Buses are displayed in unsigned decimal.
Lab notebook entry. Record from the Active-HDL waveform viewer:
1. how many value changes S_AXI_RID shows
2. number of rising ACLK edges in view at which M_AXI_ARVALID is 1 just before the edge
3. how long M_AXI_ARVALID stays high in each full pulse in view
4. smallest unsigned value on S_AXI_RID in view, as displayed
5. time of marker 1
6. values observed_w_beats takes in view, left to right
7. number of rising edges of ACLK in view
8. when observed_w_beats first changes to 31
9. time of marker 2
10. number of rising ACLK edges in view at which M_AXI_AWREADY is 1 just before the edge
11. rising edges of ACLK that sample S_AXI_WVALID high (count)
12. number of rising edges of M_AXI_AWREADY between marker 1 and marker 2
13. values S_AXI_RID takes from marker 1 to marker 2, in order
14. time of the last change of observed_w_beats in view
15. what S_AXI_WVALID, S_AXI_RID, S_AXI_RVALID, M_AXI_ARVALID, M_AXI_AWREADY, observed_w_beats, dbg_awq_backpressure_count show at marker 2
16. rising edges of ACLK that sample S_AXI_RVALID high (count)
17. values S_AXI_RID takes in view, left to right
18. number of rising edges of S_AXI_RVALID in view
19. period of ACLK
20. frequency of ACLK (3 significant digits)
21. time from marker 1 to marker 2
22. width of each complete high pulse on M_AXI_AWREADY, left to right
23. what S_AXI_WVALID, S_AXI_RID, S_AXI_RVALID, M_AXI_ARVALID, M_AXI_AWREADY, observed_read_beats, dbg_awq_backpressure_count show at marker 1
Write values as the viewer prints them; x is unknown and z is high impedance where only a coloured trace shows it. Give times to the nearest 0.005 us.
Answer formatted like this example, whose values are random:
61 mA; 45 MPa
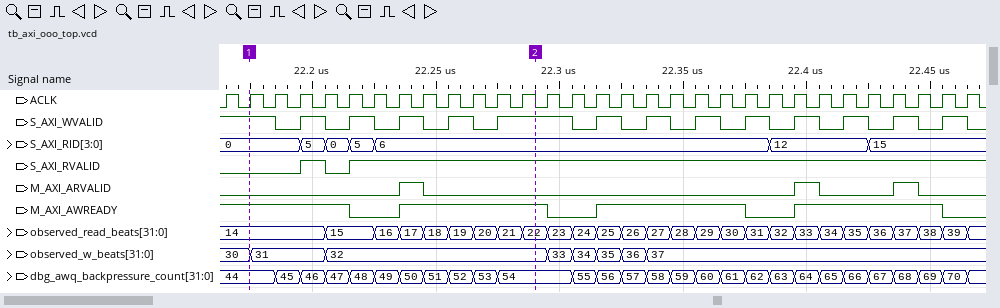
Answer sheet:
6; 3; 0.01 us, 0.01 us, 0.01 us; 0; 22.175 us; 30, 31, 32, 33, 34, 35, 36, 37; 31; 22.175 us; 22.29 us; 24; 18; 1; 0, 5, 0, 5, 6; 22.335 us; S_AXI_WVALID=1, S_AXI_RID=6, S_AXI_RVALID=1, M_AXI_ARVALID=0, M_AXI_AWREADY=1, observed_w_beats=32, dbg_awq_backpressure_count=54; 26; 0, 5, 0, 5, 6, 12, 15; 2; 0.01 us; 100 MHz; 0.115 us; 0.06 us, 0.06 us, 0.06 us; S_AXI_WVALID=1, S_AXI_RID=0, S_AXI_RVALID=0, M_AXI_ARVALID=0, M_AXI_AWREADY=1, observed_read_beats=14, dbg_awq_backpressure_count=44
